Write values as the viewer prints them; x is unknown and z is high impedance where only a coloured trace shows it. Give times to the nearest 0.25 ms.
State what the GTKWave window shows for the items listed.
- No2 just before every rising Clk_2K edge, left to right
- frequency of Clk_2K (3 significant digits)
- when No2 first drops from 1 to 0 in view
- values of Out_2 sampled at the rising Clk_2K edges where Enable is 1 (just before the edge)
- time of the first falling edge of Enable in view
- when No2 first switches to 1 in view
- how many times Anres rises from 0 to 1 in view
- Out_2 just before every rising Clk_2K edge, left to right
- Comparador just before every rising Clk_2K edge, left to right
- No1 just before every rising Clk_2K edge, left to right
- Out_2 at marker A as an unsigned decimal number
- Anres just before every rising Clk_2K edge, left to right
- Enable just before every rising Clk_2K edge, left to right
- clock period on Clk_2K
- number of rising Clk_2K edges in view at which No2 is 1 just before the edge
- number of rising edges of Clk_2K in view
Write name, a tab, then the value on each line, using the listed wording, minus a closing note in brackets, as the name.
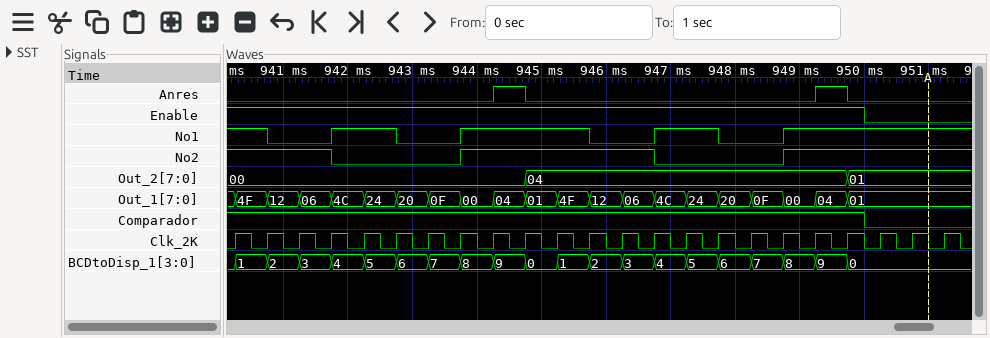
No2 just before every rising Clk_2K edge, left to right	1 1 1 1 0 0 0 0 1 1 1 1 1 1 0 0 0 0 1 1 1 1 1
frequency of Clk_2K	2.00 kHz
when No2 first drops from 1 to 0 in view	941.75 ms
values of Out_2 sampled at the rising Clk_2K edges where Enable is 1	00, 00, 00, 00, 00, 00, 00, 00, 00, 00, 04, 04, 04, 04, 04, 04, 04, 04, 04, 04
time of the first falling edge of Enable in view	950 ms
when No2 first switches to 1 in view	943.75 ms
how many times Anres rises from 0 to 1 in view	2
Out_2 just before every rising Clk_2K edge, left to right	00, 00, 00, 00, 00, 00, 00, 00, 00, 00, 04, 04, 04, 04, 04, 04, 04, 04, 04, 04, 01, 01, 01
Comparador just before every rising Clk_2K edge, left to right	1 1 1 1 1 1 1 1 1 1 1 1 1 1 1 1 1 1 1 1 0 0 0
No1 just before every rising Clk_2K edge, left to right	1 1 0 0 1 1 0 0 1 1 1 1 0 0 1 1 0 0 1 1 1 1 1
Out_2 at marker A as an unsigned decimal number	1
Anres just before every rising Clk_2K edge, left to right	0 0 0 0 0 0 0 0 0 1 0 0 0 0 0 0 0 0 0 1 0 0 0
Enable just before every rising Clk_2K edge, left to right	1 1 1 1 1 1 1 1 1 1 1 1 1 1 1 1 1 1 1 1 0 0 0
clock period on Clk_2K	0.5 ms
number of rising Clk_2K edges in view at which No2 is 1 just before the edge	15
number of rising edges of Clk_2K in view	23
